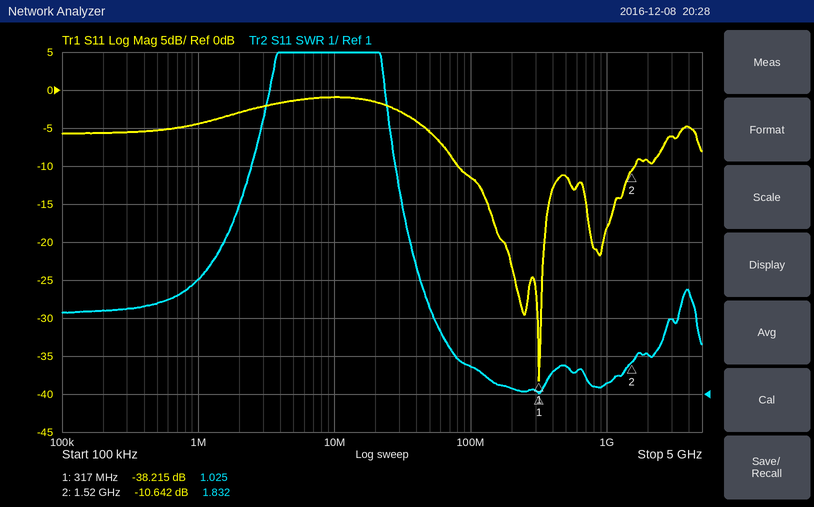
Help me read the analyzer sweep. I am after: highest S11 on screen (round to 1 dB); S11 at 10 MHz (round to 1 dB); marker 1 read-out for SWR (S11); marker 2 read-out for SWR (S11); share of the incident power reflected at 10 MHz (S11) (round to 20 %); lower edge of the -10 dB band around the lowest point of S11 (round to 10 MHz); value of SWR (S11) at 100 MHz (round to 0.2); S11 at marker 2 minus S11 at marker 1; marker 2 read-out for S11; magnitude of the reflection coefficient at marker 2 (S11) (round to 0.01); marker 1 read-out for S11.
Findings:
-1 dB
-1 dB
1.025
1.832
80 %
80 MHz
1.8
27.573 dB
-10.642 dB
0.29
-38.215 dB
